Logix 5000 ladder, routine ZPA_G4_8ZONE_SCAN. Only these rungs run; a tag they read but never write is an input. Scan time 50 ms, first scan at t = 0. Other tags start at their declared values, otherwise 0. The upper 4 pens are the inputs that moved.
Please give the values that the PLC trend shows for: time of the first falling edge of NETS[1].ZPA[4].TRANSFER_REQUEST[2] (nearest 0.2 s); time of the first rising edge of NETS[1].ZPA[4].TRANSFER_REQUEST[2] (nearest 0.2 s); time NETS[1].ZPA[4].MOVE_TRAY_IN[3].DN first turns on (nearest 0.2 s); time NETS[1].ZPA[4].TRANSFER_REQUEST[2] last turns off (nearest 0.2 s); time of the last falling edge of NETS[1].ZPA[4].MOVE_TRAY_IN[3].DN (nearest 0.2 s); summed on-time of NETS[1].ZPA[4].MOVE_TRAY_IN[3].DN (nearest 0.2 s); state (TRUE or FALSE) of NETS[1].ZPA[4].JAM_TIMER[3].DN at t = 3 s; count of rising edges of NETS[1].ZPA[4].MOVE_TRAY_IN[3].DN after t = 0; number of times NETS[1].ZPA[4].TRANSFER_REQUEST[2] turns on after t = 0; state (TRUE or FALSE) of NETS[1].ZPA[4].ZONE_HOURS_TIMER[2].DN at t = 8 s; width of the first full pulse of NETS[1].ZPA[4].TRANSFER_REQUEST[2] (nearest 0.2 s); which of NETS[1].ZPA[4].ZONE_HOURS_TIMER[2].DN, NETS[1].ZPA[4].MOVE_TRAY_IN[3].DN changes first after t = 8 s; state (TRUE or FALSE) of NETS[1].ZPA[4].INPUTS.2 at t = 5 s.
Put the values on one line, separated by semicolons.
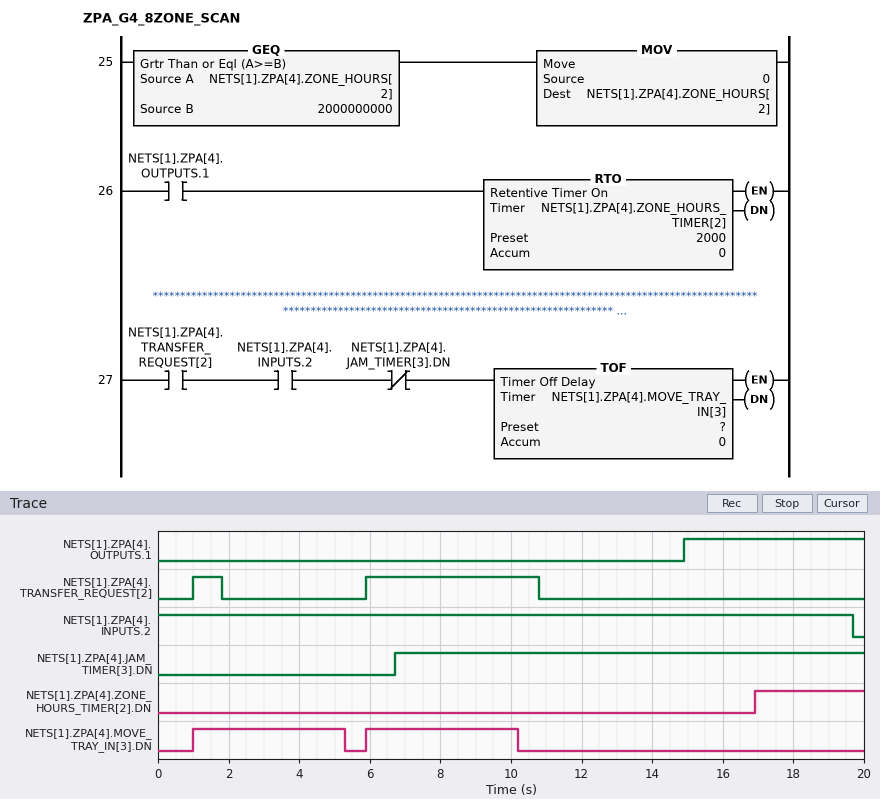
1.8 s; 1.0 s; 1.0 s; 10.8 s; 10.2 s; 8.6 s; FALSE; 2; 2; FALSE; 0.8 s; NETS[1].ZPA[4].MOVE_TRAY_IN[3].DN; TRUE
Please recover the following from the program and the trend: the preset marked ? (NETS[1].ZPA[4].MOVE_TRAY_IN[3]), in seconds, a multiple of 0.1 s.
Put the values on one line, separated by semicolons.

3.5 s
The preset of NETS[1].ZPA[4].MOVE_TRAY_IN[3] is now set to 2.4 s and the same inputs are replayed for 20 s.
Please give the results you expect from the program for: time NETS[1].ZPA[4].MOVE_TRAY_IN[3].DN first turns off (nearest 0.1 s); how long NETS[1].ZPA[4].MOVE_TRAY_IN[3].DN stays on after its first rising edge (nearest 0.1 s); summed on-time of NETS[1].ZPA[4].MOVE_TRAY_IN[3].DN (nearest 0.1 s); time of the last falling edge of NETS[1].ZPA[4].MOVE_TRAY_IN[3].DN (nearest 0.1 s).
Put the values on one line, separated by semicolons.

4.2 s; 3.2 s; 6.4 s; 9.1 s
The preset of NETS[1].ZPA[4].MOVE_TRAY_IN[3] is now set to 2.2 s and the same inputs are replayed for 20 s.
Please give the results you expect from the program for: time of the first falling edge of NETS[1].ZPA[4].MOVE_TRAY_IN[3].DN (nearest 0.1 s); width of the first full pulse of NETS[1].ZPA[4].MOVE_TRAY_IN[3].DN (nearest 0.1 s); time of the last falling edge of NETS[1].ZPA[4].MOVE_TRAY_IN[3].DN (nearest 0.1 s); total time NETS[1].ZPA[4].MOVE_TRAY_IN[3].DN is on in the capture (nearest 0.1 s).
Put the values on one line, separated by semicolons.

4.0 s; 3.0 s; 8.9 s; 6.0 s
